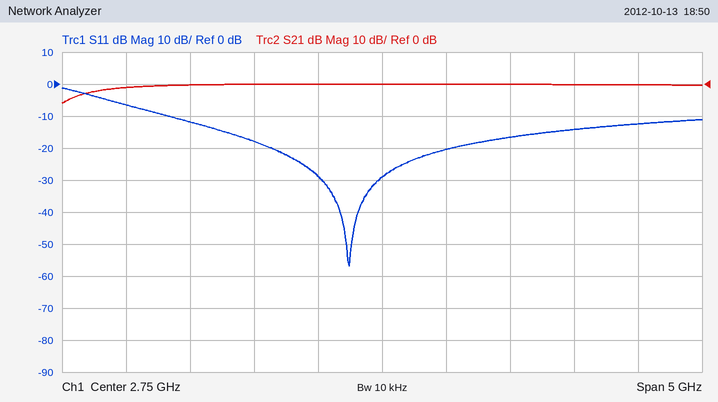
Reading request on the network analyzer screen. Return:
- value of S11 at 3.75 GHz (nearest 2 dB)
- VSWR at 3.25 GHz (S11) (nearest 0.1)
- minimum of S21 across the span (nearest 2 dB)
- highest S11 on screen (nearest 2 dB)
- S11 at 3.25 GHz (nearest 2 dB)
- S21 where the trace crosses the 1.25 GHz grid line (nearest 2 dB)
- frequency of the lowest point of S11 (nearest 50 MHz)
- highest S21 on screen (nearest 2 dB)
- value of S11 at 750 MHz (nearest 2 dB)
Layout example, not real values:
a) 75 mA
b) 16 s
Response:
a) -16 dB
b) 1.2
c) -6 dB
d) -2 dB
e) -20 dB
f) 0 dB
g) 2.50 GHz
h) 0 dB
i) -6 dB
